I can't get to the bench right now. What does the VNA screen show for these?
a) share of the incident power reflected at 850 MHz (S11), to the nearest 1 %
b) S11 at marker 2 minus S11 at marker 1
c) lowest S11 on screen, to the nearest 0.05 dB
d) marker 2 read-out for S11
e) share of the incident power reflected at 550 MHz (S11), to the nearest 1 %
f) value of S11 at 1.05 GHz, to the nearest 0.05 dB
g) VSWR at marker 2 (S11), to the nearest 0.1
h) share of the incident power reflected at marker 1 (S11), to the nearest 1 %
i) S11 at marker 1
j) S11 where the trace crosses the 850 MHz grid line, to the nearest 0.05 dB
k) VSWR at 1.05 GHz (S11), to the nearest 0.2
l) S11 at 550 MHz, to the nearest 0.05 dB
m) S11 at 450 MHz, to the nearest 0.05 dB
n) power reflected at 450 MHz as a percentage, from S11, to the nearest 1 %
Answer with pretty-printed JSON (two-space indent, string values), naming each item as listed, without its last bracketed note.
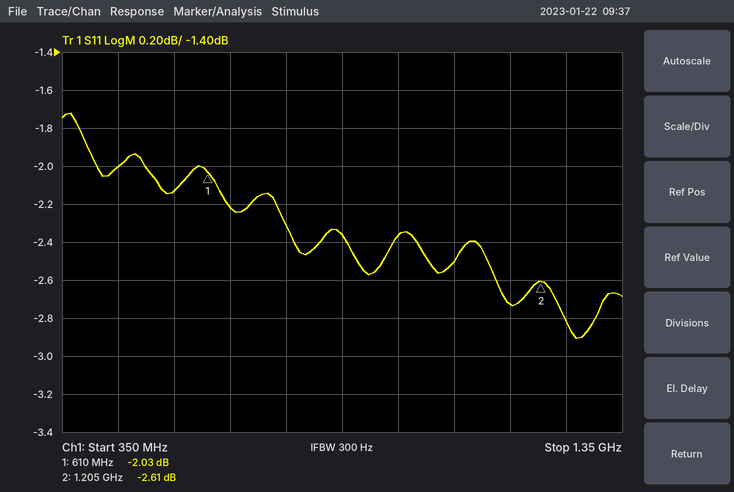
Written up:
{
  "share of the incident power reflected at 850 MHz (S11), to the nearest 1 %": "58 %",
  "S11 at marker 2 minus S11 at marker 1": "-0.58 dB",
  "lowest S11 on screen, to the nearest 0.05 dB": "-2.90 dB",
  "marker 2 read-out for S11": "-2.61 dB",
  "share of the incident power reflected at 550 MHz (S11), to the nearest 1 %": "61 %",
  "value of S11 at 1.05 GHz, to the nearest 0.05 dB": "-2.50 dB",
  "VSWR at marker 2 (S11), to the nearest 0.1": "6.7",
  "share of the incident power reflected at marker 1 (S11), to the nearest 1 %": "63 %",
  "S11 at marker 1": "-2.03 dB",
  "S11 where the trace crosses the 850 MHz grid line, to the nearest 0.05 dB": "-2.35 dB",
  "VSWR at 1.05 GHz (S11), to the nearest 0.2": "7.0",
  "S11 at 550 MHz, to the nearest 0.05 dB": "-2.15 dB",
  "S11 at 450 MHz, to the nearest 0.05 dB": "-2.00 dB",
  "power reflected at 450 MHz as a percentage, from S11, to the nearest 1 %": "63 %"
}
